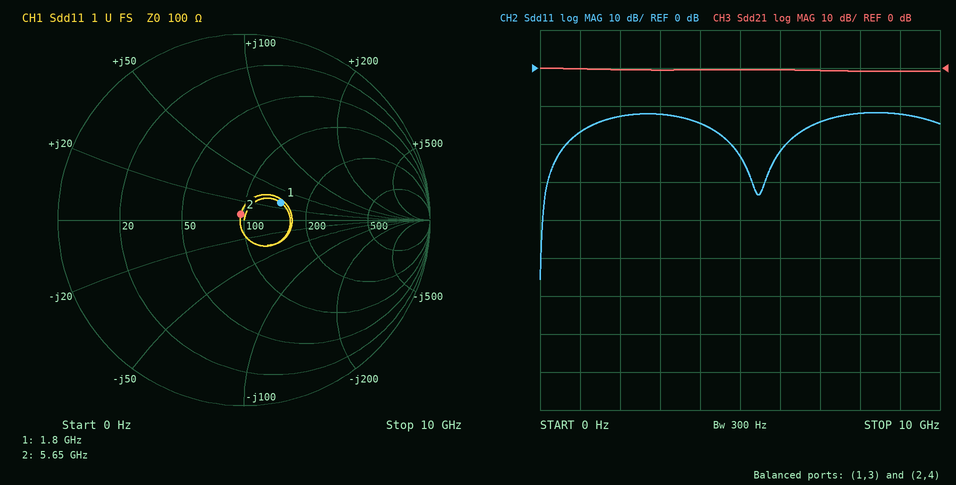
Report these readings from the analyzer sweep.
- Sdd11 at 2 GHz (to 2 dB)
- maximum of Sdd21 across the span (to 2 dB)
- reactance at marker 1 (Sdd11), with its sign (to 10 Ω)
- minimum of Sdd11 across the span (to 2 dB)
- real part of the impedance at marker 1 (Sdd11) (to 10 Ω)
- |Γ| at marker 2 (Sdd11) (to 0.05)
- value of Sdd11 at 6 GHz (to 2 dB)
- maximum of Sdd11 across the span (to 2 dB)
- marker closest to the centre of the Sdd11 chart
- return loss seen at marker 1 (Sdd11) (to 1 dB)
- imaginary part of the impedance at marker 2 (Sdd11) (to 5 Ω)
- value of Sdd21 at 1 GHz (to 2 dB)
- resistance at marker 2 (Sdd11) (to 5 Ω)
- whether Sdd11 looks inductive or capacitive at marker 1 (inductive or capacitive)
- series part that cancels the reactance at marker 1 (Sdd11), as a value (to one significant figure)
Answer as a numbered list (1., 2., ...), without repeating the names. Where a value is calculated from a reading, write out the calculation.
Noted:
1. -12 dB
2. 0 dB
3. +30 Ω
4. -56 dB
5. 150 Ω
6. 0.05
7. -22 dB
8. -12 dB
9. marker 2
10. 13 dB
11. +5 Ω
12. 0 dB
13. 95 Ω
14. inductive
15. C = 1/(2π × 1.8 GHz × 30 Ω) ≈ 3 pF
